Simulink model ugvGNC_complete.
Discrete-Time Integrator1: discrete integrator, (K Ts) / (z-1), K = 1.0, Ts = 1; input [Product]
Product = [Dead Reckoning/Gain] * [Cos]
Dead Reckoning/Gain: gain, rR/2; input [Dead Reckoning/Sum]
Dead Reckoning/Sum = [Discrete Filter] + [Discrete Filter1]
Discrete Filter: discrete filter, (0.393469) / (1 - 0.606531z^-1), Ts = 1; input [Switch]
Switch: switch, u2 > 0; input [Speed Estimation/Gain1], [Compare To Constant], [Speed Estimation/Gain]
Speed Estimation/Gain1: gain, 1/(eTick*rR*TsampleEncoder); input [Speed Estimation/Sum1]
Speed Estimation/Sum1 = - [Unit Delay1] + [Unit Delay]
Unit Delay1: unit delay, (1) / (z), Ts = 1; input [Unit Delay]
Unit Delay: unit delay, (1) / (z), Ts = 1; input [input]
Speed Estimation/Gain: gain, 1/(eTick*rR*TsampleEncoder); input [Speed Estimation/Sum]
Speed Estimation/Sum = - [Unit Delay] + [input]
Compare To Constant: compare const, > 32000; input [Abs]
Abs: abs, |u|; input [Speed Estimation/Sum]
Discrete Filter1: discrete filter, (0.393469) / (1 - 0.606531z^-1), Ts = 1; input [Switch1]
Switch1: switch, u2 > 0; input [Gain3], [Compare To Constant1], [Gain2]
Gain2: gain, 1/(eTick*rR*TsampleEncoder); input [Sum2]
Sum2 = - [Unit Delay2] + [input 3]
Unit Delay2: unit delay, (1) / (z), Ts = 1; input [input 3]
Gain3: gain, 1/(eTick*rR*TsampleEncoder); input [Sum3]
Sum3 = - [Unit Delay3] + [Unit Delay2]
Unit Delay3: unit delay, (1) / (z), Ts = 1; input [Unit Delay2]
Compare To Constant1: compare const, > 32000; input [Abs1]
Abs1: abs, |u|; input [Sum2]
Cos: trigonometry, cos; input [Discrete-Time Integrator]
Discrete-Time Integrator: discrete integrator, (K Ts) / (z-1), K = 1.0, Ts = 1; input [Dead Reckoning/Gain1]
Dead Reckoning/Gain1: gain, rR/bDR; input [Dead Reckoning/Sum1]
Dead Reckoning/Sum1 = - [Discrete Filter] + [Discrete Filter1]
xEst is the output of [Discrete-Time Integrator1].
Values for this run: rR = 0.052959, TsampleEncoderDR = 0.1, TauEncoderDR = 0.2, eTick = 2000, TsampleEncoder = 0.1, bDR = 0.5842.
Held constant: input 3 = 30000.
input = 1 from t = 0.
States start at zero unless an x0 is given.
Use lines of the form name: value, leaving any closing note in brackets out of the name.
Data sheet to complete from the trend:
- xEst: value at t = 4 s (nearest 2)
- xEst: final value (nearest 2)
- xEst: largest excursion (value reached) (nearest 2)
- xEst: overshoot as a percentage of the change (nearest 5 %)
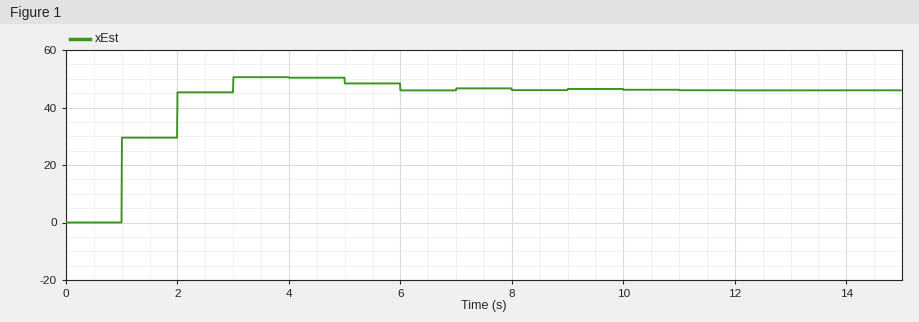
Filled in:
xEst: value at t = 4 s: 50
xEst: final value: 46
xEst: largest excursion (value reached): 50
xEst: overshoot as a percentage of the change: 10 %
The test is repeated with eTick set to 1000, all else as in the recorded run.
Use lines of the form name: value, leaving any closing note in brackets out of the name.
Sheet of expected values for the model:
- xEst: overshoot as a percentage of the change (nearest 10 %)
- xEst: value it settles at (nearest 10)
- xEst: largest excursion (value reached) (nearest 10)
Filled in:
xEst: overshoot as a percentage of the change: 50 %
xEst: value it settles at: 50
xEst: largest excursion (value reached): 80
